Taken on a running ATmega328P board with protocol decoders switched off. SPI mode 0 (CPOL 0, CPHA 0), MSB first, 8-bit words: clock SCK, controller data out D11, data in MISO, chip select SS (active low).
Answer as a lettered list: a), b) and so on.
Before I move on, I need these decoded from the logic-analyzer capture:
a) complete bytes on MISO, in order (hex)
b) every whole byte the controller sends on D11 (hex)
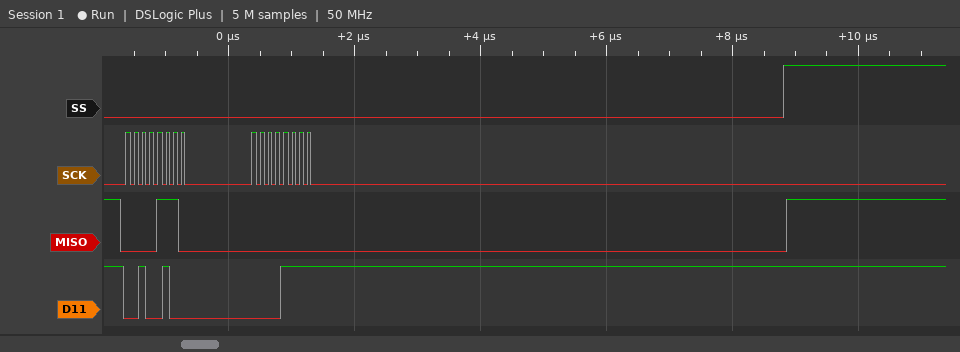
a) 0E 00
b) 24 0F
